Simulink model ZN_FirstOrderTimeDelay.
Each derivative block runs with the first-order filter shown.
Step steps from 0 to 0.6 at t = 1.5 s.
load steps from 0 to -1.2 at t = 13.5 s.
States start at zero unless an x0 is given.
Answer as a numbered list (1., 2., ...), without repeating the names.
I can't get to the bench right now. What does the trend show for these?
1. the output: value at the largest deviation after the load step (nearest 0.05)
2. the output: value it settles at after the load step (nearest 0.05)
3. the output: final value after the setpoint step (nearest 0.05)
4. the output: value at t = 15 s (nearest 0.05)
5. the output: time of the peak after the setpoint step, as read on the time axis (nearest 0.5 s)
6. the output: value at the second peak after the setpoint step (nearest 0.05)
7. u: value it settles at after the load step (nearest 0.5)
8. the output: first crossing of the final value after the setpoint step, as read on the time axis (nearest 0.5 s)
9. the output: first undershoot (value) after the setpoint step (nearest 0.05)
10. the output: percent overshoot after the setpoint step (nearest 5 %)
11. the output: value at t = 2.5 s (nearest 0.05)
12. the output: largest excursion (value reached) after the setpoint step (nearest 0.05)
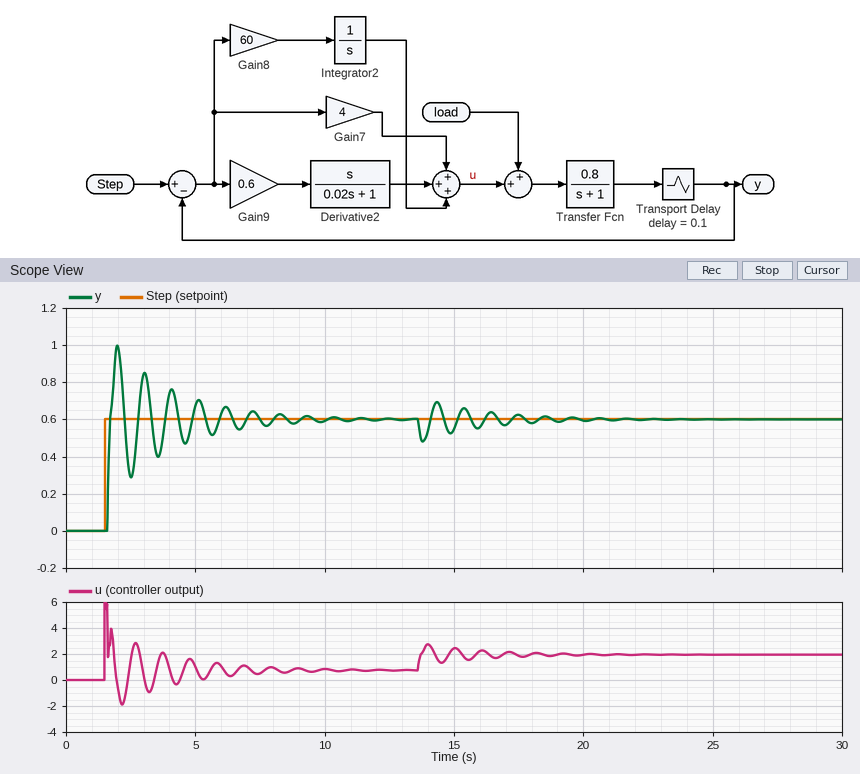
1. 0.50
2. 0.60
3. 0.60
4. 0.55
5. 2.0 s
6. 0.85
7. 2.0
8. 1.5 s
9. 0.30
10. 65 %
11. 0.30
12. 1.00
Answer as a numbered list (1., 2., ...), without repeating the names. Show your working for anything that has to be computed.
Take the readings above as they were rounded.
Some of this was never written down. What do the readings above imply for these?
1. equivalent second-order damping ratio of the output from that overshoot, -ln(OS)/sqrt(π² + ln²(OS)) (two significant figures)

1. ln(0.65) = -0.431; 0.431 / sqrt(9.870 + 0.186) = 0.14
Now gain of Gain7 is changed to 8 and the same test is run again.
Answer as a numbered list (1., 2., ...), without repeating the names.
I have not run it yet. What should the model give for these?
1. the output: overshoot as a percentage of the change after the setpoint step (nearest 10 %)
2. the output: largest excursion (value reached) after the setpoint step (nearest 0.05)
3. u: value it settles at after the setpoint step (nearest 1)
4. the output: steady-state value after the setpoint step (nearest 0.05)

1. 40 %
2. 0.85
3. 1
4. 0.60
